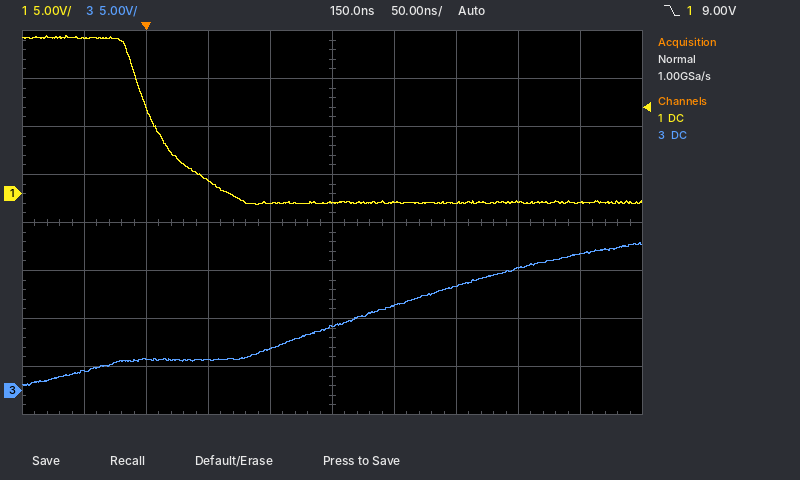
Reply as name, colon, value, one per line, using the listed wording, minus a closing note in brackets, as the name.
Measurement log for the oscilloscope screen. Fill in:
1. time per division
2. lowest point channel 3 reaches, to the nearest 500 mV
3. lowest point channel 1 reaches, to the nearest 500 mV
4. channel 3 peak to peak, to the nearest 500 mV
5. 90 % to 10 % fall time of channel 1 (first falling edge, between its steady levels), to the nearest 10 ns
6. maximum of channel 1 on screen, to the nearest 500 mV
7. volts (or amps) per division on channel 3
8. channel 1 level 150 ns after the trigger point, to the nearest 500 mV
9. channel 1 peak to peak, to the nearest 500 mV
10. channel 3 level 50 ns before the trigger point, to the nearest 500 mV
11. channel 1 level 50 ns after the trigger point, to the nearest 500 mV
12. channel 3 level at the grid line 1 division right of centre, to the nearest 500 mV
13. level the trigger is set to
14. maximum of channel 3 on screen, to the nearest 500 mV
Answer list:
time per division: 50 ns
lowest point channel 3 reaches, to the nearest 500 mV: 500 mV
lowest point channel 1 reaches, to the nearest 500 mV: -1.0 V
channel 3 peak to peak, to the nearest 500 mV: 15.0 V
90 % to 10 % fall time of channel 1 (first falling edge, between its steady levels), to the nearest 10 ns: 70 ns
maximum of channel 1 on screen, to the nearest 500 mV: 16.5 V
volts (or amps) per division on channel 3: 5 V
channel 1 level 150 ns after the trigger point, to the nearest 500 mV: -1.0 V
channel 1 peak to peak, to the nearest 500 mV: 17.5 V
channel 3 level 50 ns before the trigger point, to the nearest 500 mV: 2.0 V
channel 1 level 50 ns after the trigger point, to the nearest 500 mV: 1.5 V
channel 3 level at the grid line 1 division right of centre, to the nearest 500 mV: 9.0 V
level the trigger is set to: 9.00 V
maximum of channel 3 on screen, to the nearest 500 mV: 15.5 V
